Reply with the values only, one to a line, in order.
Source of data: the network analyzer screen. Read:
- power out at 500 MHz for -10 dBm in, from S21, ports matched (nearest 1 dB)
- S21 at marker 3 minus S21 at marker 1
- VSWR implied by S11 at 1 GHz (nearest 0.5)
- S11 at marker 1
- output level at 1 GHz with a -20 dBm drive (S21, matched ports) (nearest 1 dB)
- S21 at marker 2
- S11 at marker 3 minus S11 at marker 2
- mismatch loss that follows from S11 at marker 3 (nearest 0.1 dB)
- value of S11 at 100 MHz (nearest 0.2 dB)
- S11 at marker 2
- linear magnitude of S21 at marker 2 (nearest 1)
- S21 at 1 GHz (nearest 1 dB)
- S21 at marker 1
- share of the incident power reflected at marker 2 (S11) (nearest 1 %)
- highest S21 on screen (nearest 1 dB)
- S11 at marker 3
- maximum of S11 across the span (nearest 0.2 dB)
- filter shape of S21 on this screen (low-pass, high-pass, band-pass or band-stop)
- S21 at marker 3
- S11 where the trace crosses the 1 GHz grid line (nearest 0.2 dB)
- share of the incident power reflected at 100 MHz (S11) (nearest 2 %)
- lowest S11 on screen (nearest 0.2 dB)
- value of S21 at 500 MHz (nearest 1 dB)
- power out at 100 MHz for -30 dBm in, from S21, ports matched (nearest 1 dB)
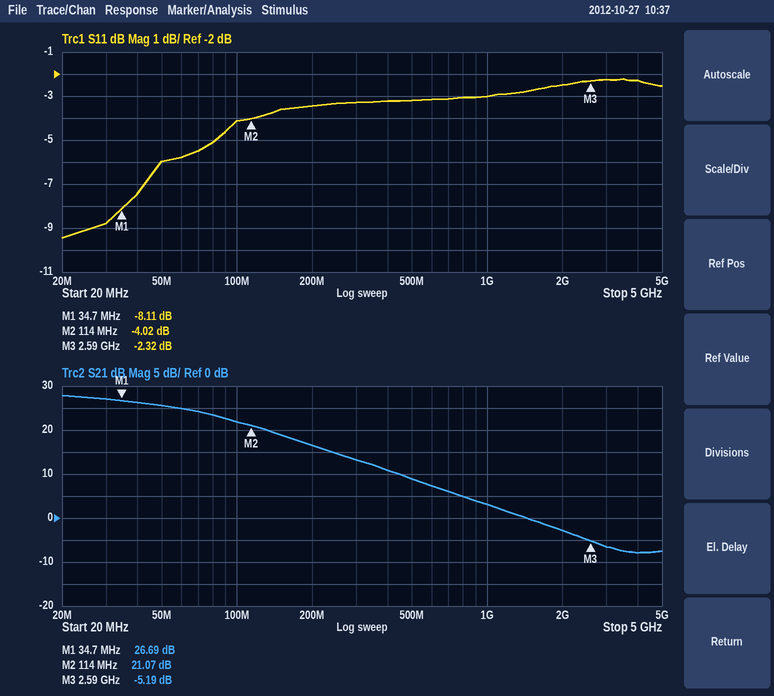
-1 dBm
-31.88 dB
6.0
-8.11 dB
-17 dBm
21.07 dB
1.70 dB
3.8 dB
-4.2 dB
-4.02 dB
11
3 dB
26.69 dB
40 %
28 dB
-2.32 dB
-2.2 dB
low-pass
-5.19 dB
-3.0 dB
38 %
-9.4 dB
9 dB
-8 dBm
